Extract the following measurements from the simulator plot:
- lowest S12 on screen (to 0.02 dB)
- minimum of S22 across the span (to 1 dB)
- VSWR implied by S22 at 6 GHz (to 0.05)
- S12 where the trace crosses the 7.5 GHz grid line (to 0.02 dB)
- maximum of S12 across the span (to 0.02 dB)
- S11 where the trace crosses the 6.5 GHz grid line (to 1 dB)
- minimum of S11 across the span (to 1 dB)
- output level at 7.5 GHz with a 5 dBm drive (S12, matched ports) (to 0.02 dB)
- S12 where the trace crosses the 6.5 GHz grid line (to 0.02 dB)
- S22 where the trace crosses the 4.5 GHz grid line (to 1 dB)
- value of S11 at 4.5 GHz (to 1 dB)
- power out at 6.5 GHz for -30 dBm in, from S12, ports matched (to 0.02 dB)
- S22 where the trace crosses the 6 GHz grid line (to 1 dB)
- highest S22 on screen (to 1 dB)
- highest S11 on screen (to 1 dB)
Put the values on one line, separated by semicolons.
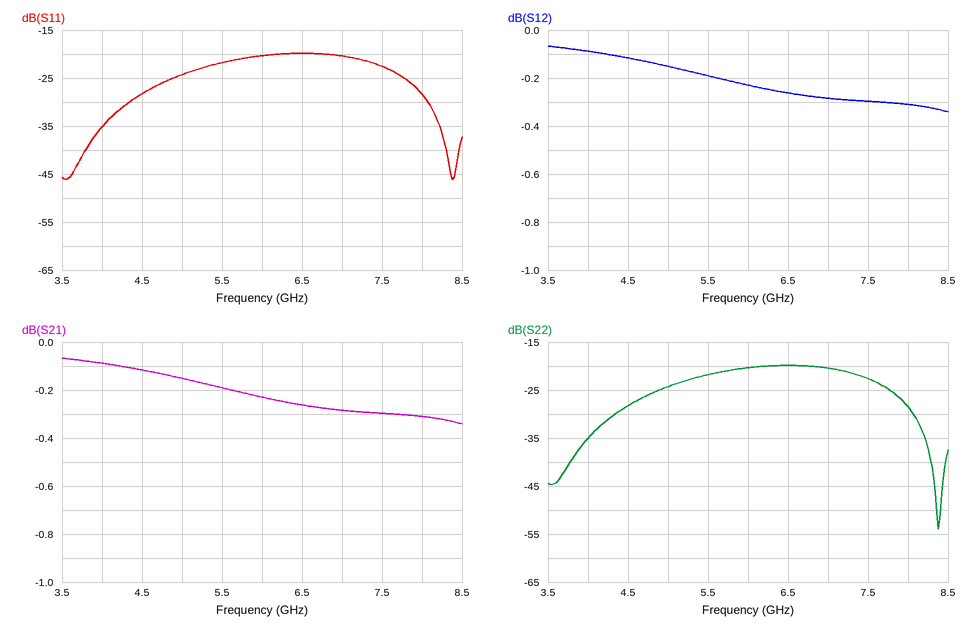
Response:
-0.34 dB; -54 dB; 1.20; -0.30 dB; -0.06 dB; -20 dB; -46 dB; 4.70 dBm; -0.26 dB; -28 dB; -28 dB; -30.26 dBm; -20 dB; -20 dB; -20 dB
